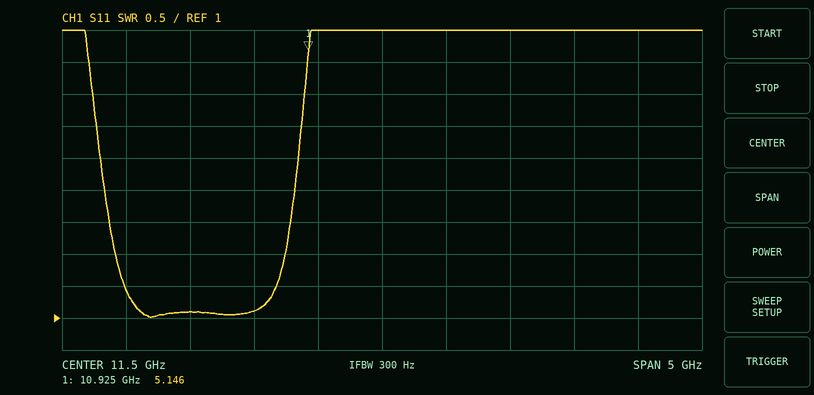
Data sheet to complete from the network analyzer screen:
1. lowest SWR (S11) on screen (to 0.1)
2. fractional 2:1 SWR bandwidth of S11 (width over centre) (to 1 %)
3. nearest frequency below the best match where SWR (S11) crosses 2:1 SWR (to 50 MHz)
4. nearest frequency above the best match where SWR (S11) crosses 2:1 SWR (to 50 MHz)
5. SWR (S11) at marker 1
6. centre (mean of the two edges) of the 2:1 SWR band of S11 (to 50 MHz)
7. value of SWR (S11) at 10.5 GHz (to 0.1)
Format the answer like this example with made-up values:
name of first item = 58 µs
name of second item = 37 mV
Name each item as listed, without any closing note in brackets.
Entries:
lowest SWR (S11) on screen = 1.0
fractional 2:1 SWR bandwidth of S11 (width over centre) = 13 %
nearest frequency below the best match where SWR (S11) crosses 2:1 SWR = 9.40 GHz
nearest frequency above the best match where SWR (S11) crosses 2:1 SWR = 10.75 GHz
SWR (S11) at marker 1 = 5.146
centre (mean of the two edges) of the 2:1 SWR band of S11 = 10.10 GHz
value of SWR (S11) at 10.5 GHz = 1.1
